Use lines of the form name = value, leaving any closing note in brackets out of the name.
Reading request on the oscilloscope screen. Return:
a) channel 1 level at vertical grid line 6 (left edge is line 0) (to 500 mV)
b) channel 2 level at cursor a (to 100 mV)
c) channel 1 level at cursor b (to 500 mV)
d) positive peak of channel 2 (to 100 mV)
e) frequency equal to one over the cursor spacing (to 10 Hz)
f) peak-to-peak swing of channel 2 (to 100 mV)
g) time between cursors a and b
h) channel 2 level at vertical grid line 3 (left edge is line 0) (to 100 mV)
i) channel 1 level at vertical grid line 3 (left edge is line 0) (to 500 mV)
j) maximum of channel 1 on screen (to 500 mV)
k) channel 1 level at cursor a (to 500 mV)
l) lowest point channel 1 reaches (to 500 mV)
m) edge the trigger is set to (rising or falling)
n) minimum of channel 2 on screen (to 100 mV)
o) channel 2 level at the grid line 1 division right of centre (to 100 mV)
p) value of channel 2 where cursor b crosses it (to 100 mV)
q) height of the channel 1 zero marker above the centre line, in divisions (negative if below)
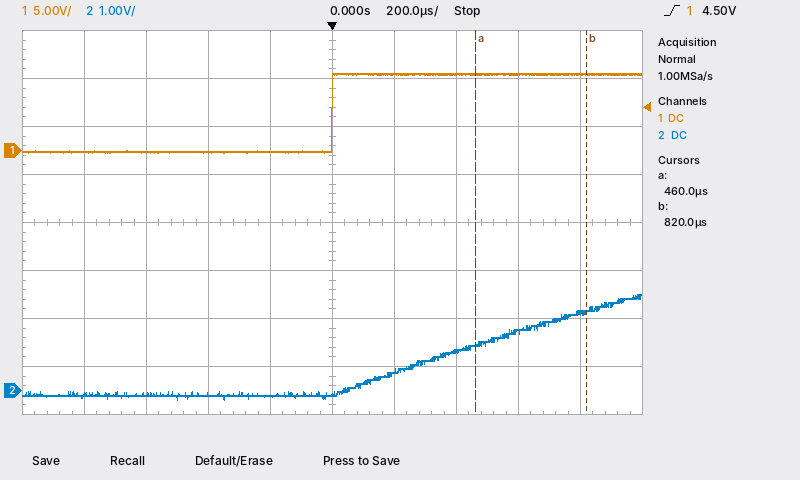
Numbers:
channel 1 level at vertical grid line 6 (left edge is line 0) = 8.0 V
channel 2 level at cursor a = 1.0 V
channel 1 level at cursor b = 8.0 V
positive peak of channel 2 = 2.0 V
frequency equal to one over the cursor spacing = 2.78 kHz
peak-to-peak swing of channel 2 = 2.2 V
time between cursors a and b = 360 µs
channel 2 level at vertical grid line 3 (left edge is line 0) = -100 mV
channel 1 level at vertical grid line 3 (left edge is line 0) = 0.0 V
maximum of channel 1 on screen = 8.0 V
channel 1 level at cursor a = 8.0 V
lowest point channel 1 reaches = 0.0 V
edge the trigger is set to = rising
minimum of channel 2 on screen = -200 mV
channel 2 level at the grid line 1 division right of centre = 400 mV
value of channel 2 where cursor b crosses it = 1.7 V
height of the channel 1 zero marker above the centre line, in divisions = +1.5 div
